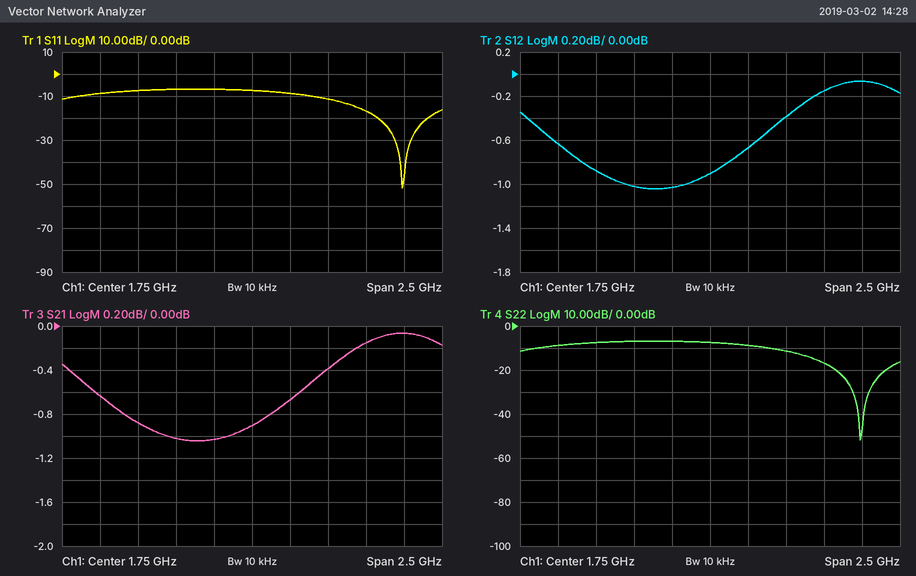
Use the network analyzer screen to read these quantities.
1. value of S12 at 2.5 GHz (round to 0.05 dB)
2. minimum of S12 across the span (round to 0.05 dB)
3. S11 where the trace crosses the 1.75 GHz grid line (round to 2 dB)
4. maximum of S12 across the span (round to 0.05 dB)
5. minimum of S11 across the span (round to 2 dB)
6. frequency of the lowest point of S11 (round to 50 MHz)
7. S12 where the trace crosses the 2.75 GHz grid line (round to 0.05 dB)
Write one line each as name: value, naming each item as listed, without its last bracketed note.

value of S12 at 2.5 GHz: -0.15 dB
minimum of S12 across the span: -1.05 dB
S11 where the trace crosses the 1.75 GHz grid line: -8 dB
maximum of S12 across the span: -0.05 dB
minimum of S11 across the span: -52 dB
frequency of the lowest point of S11: 2.75 GHz
S12 where the trace crosses the 2.75 GHz grid line: -0.05 dB
